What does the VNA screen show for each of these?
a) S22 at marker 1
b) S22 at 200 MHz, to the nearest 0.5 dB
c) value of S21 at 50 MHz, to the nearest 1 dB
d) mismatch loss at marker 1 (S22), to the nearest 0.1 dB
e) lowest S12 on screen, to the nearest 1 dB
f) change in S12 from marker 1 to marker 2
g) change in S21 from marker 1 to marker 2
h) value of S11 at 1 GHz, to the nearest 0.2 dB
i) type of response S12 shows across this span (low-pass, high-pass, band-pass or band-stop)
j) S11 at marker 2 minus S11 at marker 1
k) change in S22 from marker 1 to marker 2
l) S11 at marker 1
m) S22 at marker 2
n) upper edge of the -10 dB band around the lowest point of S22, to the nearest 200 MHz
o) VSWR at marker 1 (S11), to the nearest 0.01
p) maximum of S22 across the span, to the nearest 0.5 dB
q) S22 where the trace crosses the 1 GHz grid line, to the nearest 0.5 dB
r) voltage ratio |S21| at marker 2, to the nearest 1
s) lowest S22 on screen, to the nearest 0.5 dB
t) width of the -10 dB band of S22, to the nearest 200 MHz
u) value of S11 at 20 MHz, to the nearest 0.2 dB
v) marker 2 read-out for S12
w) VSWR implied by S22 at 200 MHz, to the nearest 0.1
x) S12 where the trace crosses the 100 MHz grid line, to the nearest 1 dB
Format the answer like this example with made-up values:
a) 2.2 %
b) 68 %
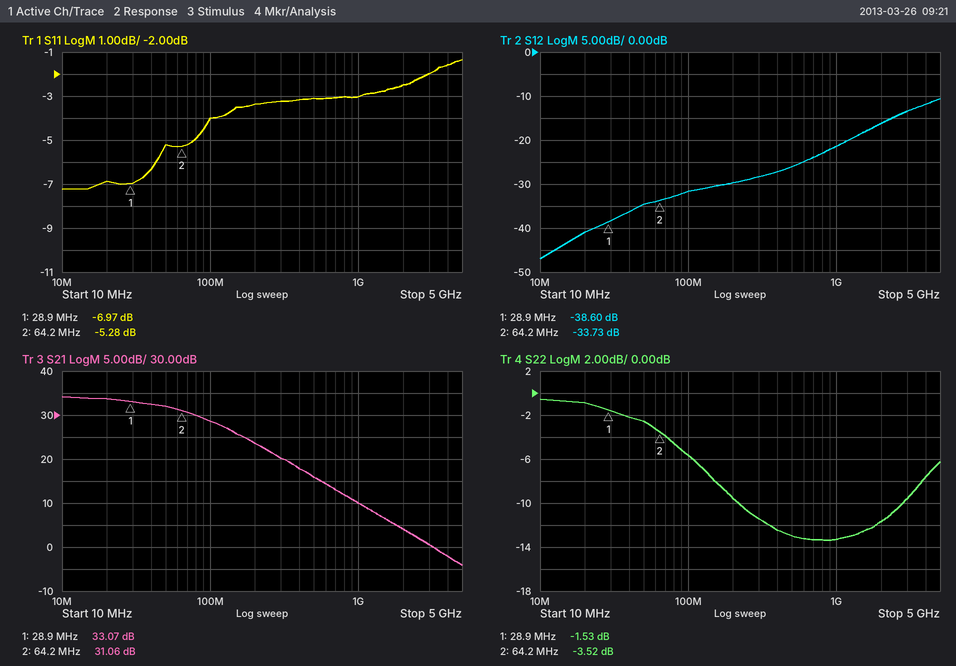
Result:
a) -1.53 dB
b) -9.5 dB
c) 32 dB
d) 5.3 dB
e) -47 dB
f) 4.87 dB
g) -2.01 dB
h) -3.0 dB
i) high-pass
j) 1.69 dB
k) -1.99 dB
l) -6.97 dB
m) -3.52 dB
n) 2.8 GHz
o) 2.62
p) -0.5 dB
q) -13.5 dB
r) 36
s) -13.5 dB
t) 2.6 GHz
u) -6.8 dB
v) -33.73 dB
w) 2.0
x) -32 dB
